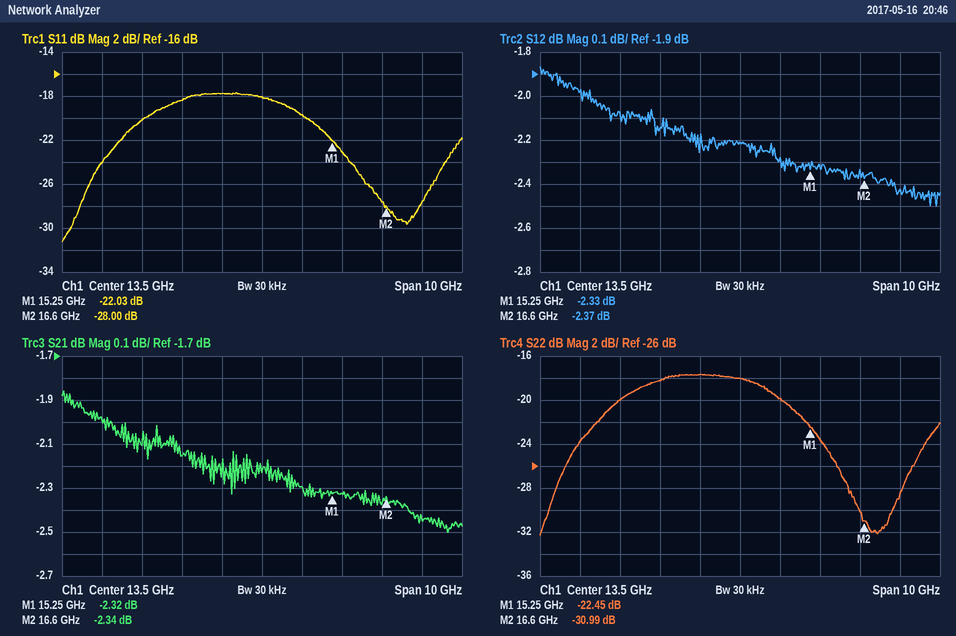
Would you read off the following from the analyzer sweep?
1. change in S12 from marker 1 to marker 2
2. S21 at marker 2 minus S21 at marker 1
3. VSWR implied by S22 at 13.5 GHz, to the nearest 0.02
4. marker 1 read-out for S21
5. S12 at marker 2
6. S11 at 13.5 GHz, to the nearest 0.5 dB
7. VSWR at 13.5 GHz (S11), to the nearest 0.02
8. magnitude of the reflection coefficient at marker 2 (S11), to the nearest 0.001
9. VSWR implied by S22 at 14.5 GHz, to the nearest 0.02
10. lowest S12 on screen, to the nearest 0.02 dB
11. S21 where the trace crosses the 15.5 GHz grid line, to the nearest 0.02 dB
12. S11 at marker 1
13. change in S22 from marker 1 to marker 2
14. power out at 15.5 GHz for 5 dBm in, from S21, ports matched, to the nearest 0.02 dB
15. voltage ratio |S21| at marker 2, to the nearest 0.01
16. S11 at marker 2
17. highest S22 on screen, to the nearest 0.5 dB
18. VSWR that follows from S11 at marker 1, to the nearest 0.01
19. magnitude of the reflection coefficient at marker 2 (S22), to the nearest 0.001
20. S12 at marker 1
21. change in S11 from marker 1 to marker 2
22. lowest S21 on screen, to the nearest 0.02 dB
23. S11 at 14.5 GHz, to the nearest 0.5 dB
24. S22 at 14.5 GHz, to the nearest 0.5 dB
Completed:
-0.04 dB
-0.02 dB
1.28
-2.32 dB
-2.37 dB
-18.0 dB
1.28
0.040
1.22
-2.50 dB
-2.32 dB
-22.03 dB
-8.54 dB
2.68 dBm
0.76
-28.00 dB
-17.5 dB
1.17
0.028
-2.33 dB
-5.97 dB
-2.50 dB
-19.5 dB
-20.0 dB
